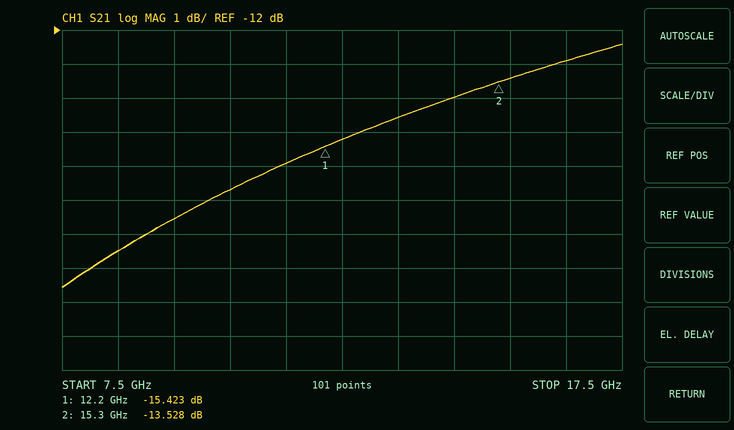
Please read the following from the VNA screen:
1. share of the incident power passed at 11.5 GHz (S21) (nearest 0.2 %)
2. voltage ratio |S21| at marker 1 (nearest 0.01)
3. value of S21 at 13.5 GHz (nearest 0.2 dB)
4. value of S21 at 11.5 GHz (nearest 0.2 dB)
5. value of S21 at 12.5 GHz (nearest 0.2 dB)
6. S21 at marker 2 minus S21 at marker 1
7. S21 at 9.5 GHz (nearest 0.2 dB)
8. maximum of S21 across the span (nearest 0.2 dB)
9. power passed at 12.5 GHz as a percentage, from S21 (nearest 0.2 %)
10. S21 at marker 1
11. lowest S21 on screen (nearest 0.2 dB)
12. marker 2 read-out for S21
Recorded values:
2.6 %
0.17
-14.6 dB
-16.0 dB
-15.2 dB
1.895 dB
-17.6 dB
-12.4 dB
3.0 %
-15.423 dB
-19.6 dB
-13.528 dB
